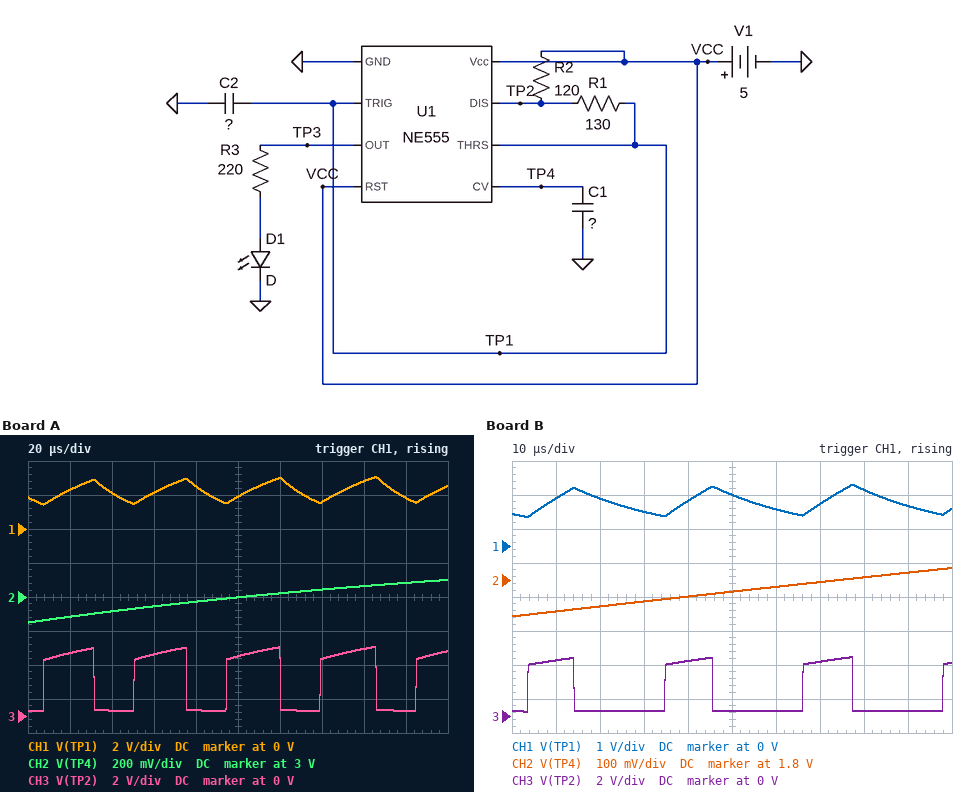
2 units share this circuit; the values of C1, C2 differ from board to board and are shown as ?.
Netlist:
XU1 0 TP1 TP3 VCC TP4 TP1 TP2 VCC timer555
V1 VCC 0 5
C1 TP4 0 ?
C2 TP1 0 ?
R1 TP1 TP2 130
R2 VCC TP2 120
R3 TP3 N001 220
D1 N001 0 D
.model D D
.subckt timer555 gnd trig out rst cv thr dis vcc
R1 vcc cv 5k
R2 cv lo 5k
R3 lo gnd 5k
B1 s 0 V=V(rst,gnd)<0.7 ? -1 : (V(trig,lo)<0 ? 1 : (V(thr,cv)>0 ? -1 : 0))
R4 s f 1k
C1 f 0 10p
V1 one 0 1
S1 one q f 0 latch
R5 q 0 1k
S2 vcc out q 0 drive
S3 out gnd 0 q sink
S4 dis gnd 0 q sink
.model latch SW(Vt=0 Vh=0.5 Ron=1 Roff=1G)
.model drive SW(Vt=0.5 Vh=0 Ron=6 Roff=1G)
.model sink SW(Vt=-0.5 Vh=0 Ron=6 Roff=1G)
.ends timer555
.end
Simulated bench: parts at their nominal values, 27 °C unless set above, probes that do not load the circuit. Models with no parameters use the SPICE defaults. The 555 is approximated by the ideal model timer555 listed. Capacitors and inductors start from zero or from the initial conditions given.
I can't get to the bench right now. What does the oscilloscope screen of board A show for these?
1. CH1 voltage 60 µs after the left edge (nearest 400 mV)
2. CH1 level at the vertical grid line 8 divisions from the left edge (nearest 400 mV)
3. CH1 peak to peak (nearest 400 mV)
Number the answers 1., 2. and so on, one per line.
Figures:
1. 2.0 V
2. 2.8 V
3. 1.6 V
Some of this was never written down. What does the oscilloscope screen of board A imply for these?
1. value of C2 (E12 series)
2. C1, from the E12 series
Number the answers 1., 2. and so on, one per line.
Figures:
1. 180 nF
2. 82 nF
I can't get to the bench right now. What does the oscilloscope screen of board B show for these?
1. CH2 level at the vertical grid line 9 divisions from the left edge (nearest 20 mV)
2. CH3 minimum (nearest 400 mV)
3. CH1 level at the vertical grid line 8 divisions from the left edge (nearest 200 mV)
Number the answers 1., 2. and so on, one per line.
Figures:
1. 1.82 V
2. 400 mV
3. 1.6 V
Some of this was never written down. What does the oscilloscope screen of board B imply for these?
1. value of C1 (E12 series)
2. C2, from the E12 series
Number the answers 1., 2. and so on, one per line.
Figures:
1. 330 nF
2. 180 nF
